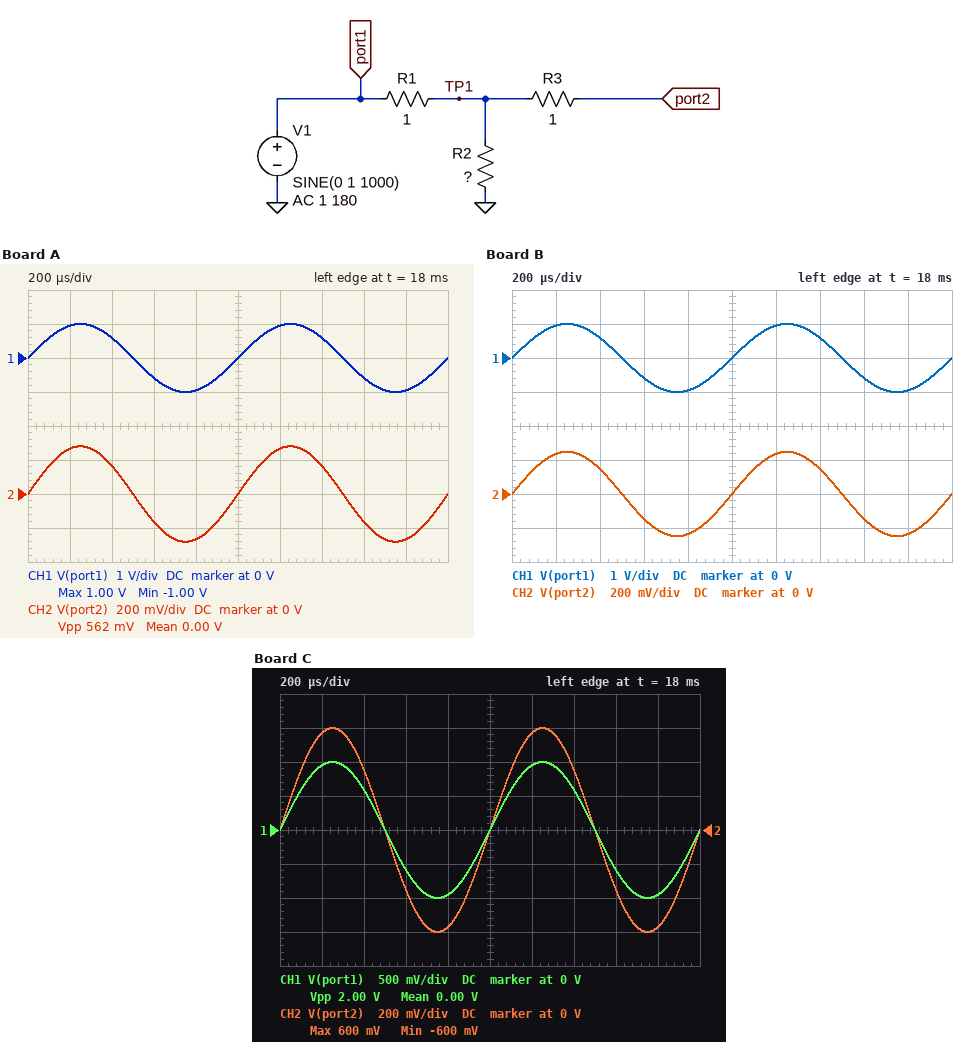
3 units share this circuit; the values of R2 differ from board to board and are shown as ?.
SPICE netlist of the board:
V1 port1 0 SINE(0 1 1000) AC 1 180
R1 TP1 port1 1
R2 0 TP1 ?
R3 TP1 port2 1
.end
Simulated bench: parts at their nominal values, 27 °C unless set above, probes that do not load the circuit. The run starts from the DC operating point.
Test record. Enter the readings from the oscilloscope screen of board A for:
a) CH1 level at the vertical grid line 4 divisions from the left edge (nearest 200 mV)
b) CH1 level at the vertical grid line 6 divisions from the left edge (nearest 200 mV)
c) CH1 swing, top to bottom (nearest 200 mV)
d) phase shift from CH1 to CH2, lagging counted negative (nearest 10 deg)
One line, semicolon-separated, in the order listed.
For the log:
-1.0 V; 1.0 V; 2.0 V; 0 deg
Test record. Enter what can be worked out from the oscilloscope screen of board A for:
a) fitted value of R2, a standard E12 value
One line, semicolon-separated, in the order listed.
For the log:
0.39 Ω
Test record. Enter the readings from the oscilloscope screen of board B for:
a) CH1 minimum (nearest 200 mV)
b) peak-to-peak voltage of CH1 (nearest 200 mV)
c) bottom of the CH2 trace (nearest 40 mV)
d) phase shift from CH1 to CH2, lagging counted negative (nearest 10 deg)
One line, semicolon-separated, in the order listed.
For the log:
-1.0 V; 2.0 V; -240 mV; 0 deg
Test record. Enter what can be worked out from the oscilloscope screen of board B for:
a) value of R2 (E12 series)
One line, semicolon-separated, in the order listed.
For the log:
0.33 Ω
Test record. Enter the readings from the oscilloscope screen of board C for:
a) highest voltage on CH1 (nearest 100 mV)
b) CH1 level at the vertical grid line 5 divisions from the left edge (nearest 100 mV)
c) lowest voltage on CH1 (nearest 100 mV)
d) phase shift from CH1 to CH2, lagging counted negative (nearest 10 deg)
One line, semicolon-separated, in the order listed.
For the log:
1.0 V; 0 V; -1.0 V; 0 deg
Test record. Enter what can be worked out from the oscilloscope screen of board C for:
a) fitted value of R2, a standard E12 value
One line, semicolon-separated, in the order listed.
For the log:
1.5 Ω
